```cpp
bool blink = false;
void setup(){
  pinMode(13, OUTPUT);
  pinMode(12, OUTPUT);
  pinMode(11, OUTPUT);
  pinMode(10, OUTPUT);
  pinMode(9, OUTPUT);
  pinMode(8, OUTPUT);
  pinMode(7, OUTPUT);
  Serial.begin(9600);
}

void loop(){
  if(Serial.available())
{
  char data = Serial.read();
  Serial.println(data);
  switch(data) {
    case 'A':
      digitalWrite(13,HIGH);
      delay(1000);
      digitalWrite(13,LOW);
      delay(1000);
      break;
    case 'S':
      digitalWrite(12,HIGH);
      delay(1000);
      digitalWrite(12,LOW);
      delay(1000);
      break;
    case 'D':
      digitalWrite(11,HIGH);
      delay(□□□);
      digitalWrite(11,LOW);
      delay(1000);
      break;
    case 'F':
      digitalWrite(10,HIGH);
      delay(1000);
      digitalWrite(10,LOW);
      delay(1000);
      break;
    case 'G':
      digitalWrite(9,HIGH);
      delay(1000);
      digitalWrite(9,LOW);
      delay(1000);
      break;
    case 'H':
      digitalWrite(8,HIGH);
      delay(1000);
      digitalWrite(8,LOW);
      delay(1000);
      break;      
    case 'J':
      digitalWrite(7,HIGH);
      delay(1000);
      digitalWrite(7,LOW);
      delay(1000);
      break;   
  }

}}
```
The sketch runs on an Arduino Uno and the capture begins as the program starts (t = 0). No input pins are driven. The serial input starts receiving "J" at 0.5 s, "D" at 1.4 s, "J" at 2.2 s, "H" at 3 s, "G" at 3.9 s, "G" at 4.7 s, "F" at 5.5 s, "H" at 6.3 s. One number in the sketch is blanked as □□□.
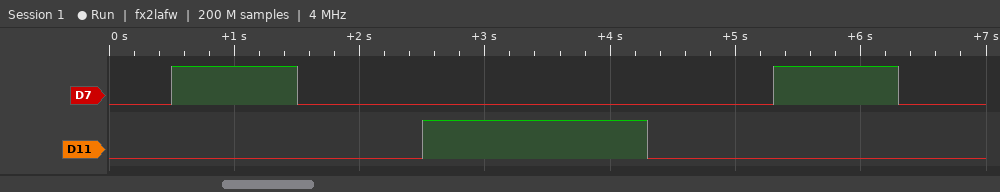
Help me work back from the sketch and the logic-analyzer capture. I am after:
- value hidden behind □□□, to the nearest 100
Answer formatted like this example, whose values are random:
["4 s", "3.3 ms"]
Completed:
["1800"]
